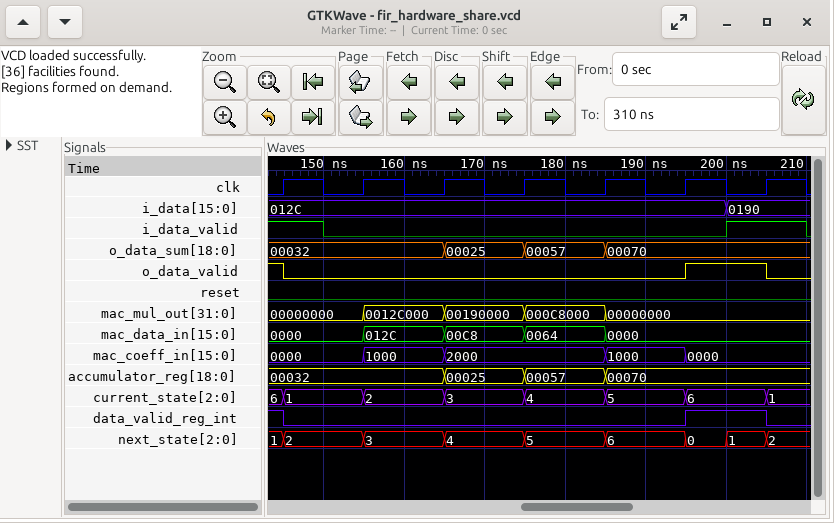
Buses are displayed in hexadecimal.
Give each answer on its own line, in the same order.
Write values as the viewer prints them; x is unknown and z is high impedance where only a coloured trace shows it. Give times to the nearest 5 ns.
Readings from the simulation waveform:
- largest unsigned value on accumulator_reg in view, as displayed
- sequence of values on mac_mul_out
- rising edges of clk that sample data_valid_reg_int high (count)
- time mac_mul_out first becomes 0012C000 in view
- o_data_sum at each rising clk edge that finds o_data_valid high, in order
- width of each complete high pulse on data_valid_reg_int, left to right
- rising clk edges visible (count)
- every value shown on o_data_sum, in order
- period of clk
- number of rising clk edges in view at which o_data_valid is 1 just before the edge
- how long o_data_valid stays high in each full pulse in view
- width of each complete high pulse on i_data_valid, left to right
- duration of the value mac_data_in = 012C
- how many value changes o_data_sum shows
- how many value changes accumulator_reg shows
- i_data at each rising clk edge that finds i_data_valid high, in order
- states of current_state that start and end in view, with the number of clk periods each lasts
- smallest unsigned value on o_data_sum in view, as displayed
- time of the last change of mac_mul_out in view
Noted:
00070
00000000, 0012C000, 00190000, 000C8000, 00000000
2
155 ns
00032, 00070
10 ns
7
00032, 00025, 00057, 00070
10 ns
2
10 ns
10 ns
10 ns
3
3
012C, 0190
1: 1, 2: 1, 3: 1, 4: 1, 5: 1, 6: 1
00025
185 ns
